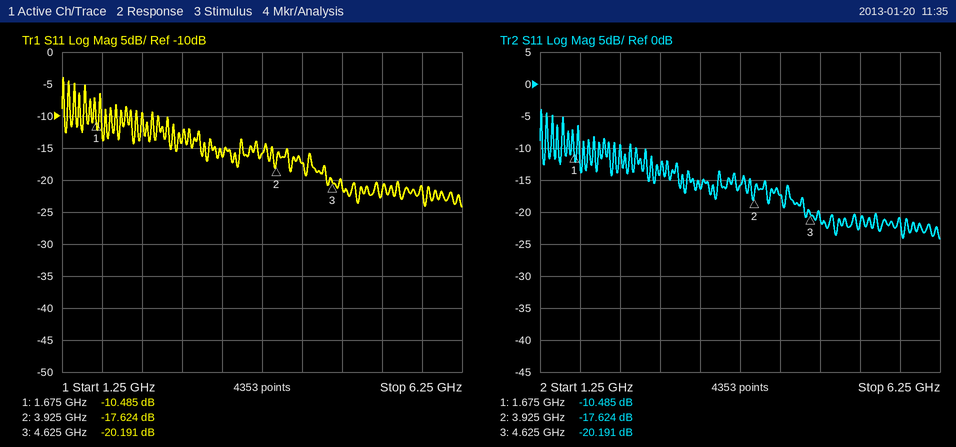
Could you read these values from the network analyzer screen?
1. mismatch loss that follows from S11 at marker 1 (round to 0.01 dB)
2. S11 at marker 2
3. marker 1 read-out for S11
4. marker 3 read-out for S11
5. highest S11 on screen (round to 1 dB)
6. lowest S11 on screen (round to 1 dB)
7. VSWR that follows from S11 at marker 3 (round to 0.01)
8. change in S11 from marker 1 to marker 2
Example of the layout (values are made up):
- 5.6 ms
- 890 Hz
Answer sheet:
- 0.41 dB
- -17.624 dB
- -10.485 dB
- -20.191 dB
- -4 dB
- -24 dB
- 1.22
- -7.139 dB
